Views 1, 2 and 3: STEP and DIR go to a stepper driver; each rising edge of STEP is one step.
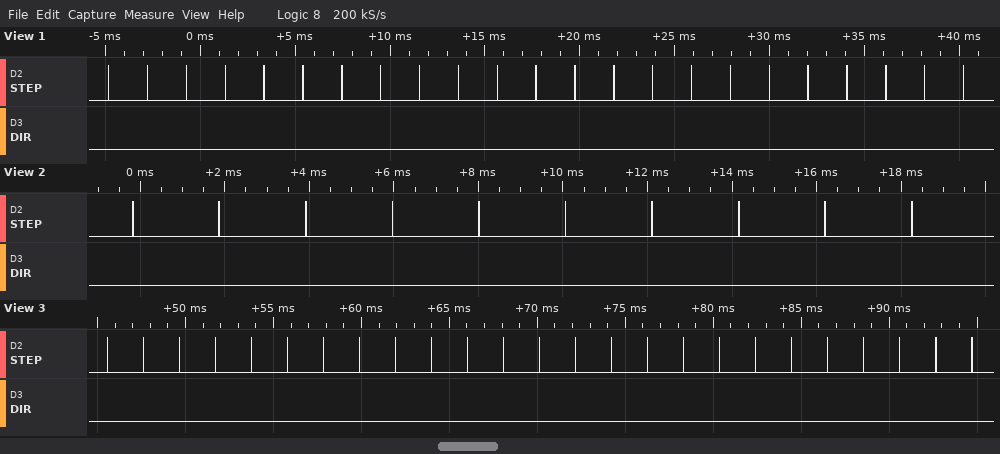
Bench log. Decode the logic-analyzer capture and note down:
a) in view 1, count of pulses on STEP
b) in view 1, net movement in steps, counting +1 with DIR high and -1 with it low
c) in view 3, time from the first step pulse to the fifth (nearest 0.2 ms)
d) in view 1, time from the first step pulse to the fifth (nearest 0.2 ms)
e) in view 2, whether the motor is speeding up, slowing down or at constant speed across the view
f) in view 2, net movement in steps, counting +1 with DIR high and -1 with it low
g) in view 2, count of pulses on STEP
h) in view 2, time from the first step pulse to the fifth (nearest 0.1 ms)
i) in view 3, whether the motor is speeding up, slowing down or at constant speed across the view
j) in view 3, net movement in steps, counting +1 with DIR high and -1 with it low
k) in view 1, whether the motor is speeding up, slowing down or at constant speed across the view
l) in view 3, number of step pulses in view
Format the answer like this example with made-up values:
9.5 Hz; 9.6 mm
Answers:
23; -23; 8.2 ms; 8.2 ms; constant speed; -10; 10; 8.2 ms; constant speed; -25; constant speed; 25
